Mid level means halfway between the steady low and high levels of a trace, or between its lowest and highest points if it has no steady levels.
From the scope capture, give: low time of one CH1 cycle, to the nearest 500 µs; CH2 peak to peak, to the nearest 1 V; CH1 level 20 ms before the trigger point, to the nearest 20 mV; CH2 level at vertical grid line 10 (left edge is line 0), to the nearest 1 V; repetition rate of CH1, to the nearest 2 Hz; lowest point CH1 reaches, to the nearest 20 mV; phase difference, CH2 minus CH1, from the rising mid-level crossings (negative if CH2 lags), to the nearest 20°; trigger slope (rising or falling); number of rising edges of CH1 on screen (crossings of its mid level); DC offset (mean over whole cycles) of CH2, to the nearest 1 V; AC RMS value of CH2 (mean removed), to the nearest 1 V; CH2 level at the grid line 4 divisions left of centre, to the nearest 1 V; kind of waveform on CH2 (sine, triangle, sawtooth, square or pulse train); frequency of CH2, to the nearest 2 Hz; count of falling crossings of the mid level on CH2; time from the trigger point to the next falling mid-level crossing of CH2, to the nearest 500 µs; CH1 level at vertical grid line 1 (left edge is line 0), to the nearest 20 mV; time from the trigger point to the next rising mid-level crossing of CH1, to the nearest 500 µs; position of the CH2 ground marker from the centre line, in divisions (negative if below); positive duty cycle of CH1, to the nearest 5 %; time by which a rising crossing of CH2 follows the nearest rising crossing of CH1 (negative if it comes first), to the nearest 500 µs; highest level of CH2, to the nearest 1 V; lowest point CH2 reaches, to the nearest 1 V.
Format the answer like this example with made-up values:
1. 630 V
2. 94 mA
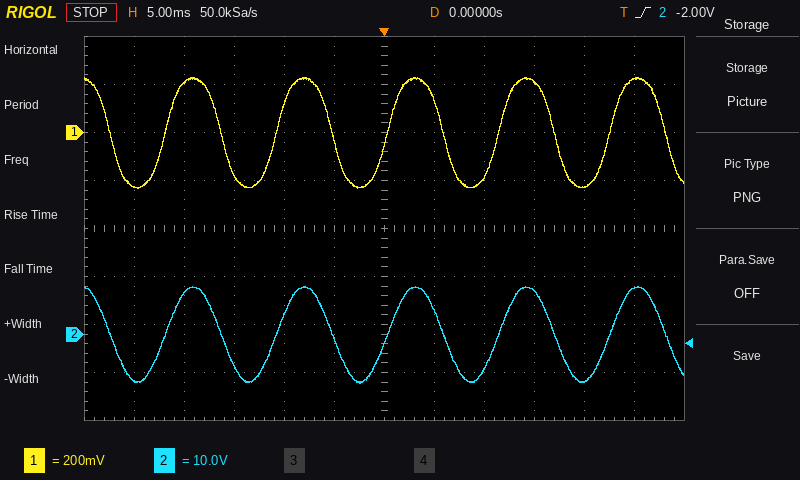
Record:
1. 5.5 ms
2. 20 V
3. 200 mV
4. -10 V
5. 90 Hz
6. -240 mV
7. 0°
8. rising
9. 5
10. 0 V
11. 7 V
12. 8 V
13. sine
14. 90 Hz
15. 6
16. 6.0 ms
17. -220 mV
18. 500 µs
19. -2.2 div
20. 50 %
21. 0.0 ms
22. 10 V
23. -10 V
